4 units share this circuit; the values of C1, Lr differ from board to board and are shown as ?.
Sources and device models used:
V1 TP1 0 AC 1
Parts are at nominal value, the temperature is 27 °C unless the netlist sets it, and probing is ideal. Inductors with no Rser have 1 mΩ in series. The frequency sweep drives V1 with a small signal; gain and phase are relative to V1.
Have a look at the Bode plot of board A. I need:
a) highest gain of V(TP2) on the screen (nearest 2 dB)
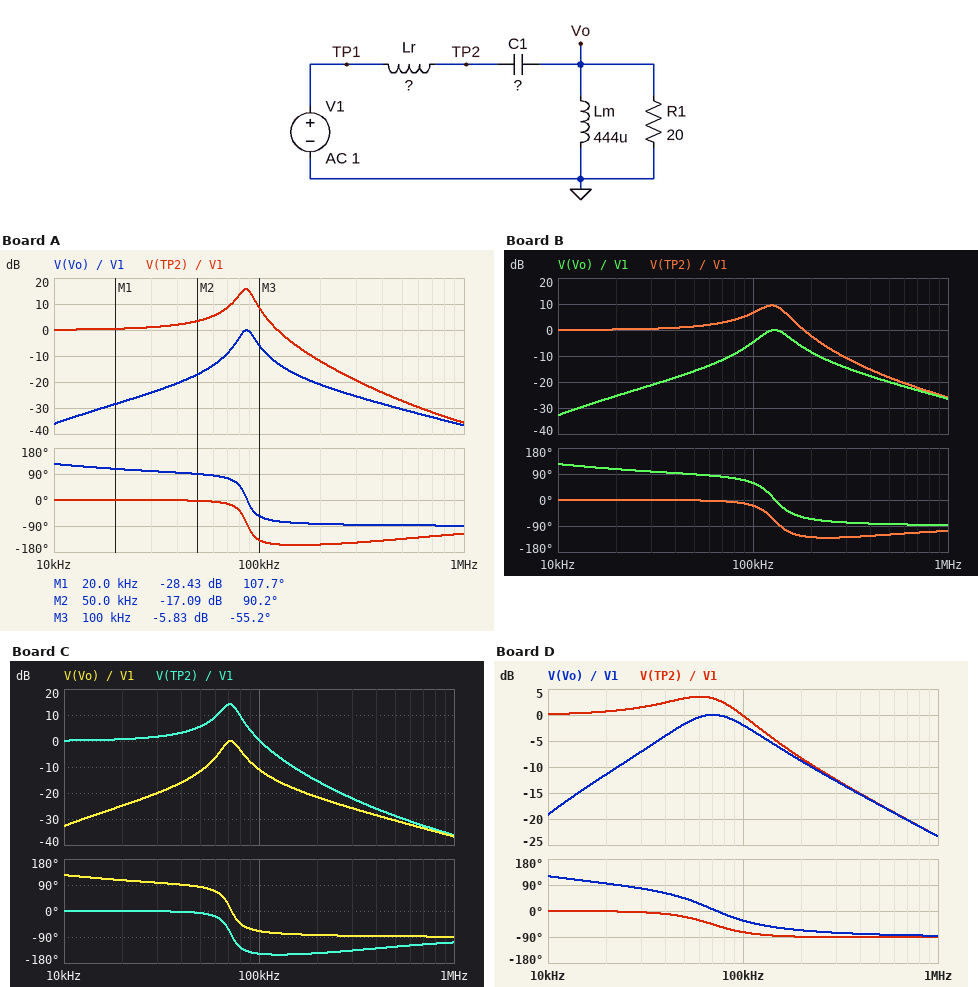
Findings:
16 dB
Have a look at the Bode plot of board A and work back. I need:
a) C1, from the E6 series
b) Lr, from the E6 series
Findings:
15 nF
220 µH
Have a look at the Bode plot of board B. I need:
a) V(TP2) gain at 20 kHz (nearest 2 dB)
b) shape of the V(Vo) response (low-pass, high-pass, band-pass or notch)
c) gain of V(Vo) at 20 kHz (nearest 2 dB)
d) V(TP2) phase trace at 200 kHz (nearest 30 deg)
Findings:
0 dB
band-pass
-26 dB
-120 deg
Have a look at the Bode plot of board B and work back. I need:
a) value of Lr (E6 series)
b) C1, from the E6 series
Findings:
68 µH
22 nF
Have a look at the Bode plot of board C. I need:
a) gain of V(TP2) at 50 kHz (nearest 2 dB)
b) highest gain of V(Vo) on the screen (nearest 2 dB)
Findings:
6 dB
0 dB
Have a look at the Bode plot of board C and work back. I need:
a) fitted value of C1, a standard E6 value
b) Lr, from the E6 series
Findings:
22 nF
220 µH
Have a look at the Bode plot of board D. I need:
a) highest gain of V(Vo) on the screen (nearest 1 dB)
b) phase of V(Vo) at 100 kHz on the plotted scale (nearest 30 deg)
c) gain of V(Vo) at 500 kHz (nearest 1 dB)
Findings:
0 dB
-30 deg
-17 dB
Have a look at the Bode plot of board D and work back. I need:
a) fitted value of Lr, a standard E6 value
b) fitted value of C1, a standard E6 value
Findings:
47 µH
100 nF
